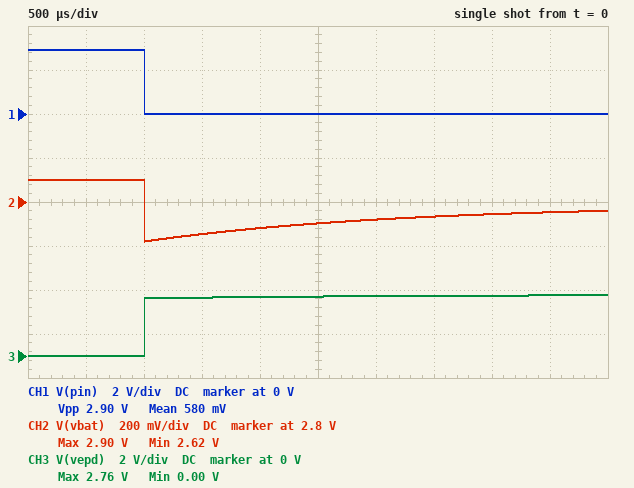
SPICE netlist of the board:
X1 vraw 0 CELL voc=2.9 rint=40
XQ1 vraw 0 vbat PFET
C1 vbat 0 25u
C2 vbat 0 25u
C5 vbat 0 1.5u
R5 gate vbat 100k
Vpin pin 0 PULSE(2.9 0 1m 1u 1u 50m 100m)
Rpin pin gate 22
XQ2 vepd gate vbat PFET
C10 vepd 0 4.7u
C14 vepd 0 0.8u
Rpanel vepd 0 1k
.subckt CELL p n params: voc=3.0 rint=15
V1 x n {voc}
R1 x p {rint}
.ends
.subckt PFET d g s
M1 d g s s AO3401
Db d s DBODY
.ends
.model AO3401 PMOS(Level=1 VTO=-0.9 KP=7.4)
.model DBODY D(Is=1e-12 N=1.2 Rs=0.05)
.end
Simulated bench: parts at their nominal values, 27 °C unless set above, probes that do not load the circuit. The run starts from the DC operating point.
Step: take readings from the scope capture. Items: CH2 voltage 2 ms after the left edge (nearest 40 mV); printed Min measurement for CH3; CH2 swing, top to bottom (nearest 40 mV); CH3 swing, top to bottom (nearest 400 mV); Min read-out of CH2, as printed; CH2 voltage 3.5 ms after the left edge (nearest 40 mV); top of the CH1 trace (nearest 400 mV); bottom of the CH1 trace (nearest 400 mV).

2.68 V
0.00 V
280 mV
2.8 V
2.62 V
2.72 V
2.8 V
0 V
